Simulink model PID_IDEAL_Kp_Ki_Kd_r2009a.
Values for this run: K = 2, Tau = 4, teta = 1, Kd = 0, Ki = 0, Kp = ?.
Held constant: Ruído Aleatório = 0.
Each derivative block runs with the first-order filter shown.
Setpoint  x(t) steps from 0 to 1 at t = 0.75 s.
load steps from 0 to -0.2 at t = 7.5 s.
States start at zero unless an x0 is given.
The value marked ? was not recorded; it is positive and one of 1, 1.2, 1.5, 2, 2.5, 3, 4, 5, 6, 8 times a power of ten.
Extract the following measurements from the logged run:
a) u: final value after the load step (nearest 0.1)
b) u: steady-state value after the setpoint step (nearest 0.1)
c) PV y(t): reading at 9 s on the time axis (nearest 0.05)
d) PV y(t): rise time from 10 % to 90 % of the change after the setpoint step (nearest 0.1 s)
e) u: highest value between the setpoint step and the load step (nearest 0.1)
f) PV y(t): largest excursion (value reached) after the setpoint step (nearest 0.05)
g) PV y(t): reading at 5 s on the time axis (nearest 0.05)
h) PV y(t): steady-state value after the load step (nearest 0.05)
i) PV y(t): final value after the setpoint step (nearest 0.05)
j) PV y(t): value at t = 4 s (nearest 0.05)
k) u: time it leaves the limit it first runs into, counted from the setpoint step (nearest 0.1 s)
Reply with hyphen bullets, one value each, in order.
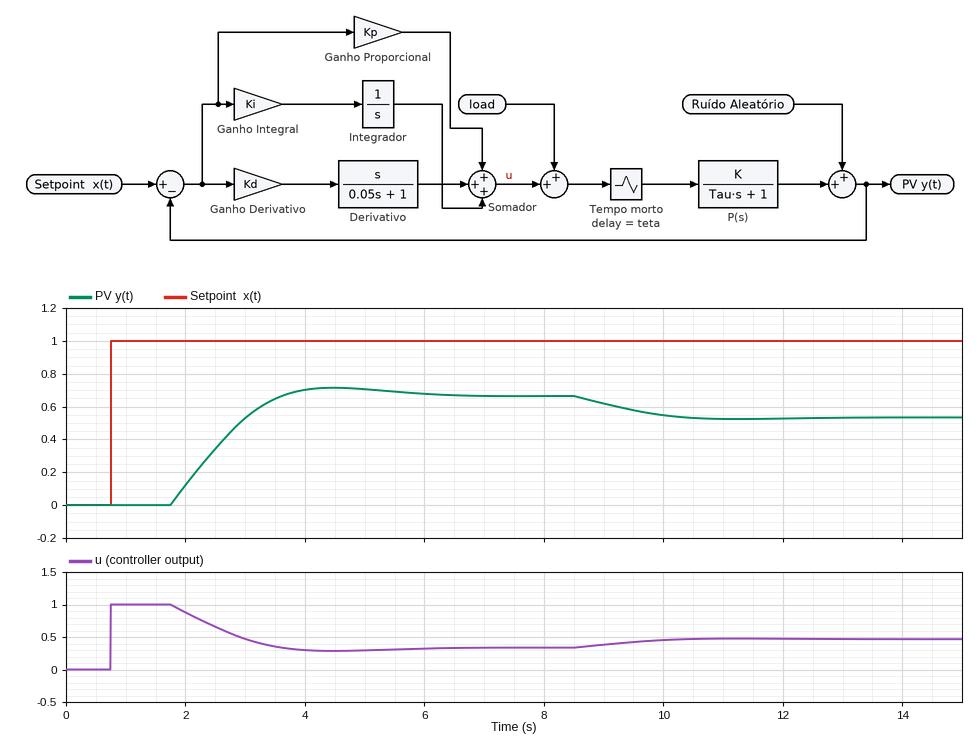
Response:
- 0.5
- 0.3
- 0.60
- 1.4 s
- 1.0
- 0.70
- 0.70
- 0.55
- 0.65
- 0.70
- 1.0 s
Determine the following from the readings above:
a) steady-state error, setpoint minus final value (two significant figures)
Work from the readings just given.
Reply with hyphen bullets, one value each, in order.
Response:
- 0.35
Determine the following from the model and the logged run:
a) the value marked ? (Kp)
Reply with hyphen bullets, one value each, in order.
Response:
- 1
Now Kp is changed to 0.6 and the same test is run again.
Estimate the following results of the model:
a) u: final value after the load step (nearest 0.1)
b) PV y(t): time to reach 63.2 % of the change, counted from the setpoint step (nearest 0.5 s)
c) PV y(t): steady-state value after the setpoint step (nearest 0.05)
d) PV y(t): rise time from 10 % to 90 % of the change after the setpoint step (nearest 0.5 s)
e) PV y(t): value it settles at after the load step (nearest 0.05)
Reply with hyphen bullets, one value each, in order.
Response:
- 0.4
- 2.5 s
- 0.55
- 2.5 s
- 0.35
